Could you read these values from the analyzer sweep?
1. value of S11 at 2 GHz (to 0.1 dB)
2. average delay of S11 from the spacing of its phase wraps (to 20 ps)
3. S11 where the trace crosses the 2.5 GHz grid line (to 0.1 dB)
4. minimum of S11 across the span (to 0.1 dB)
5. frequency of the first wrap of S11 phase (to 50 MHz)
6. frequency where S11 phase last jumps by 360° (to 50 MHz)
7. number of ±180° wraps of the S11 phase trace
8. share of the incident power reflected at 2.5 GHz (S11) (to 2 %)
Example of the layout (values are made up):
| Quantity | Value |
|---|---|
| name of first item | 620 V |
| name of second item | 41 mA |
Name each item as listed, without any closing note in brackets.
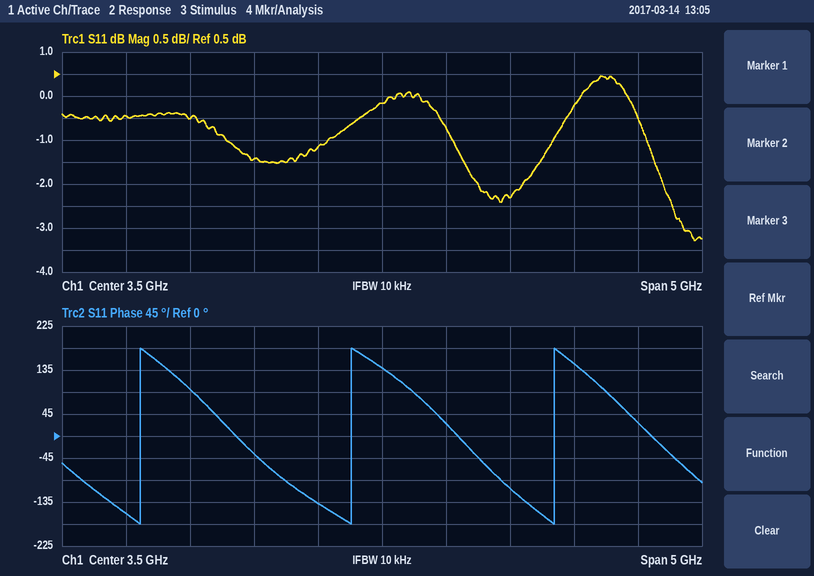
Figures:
| Quantity | Value |
|---|---|
| value of S11 at 2 GHz | -0.5 dB |
| average delay of S11 from the spacing of its phase wraps | 620 ps |
| S11 where the trace crosses the 2.5 GHz grid line | -1.4 dB |
| minimum of S11 across the span | -3.3 dB |
| frequency of the first wrap of S11 phase | 1.60 GHz |
| frequency where S11 phase last jumps by 360° | 4.85 GHz |
| number of ±180° wraps of the S11 phase trace | 3 |
| share of the incident power reflected at 2.5 GHz (S11) | 72 % |
